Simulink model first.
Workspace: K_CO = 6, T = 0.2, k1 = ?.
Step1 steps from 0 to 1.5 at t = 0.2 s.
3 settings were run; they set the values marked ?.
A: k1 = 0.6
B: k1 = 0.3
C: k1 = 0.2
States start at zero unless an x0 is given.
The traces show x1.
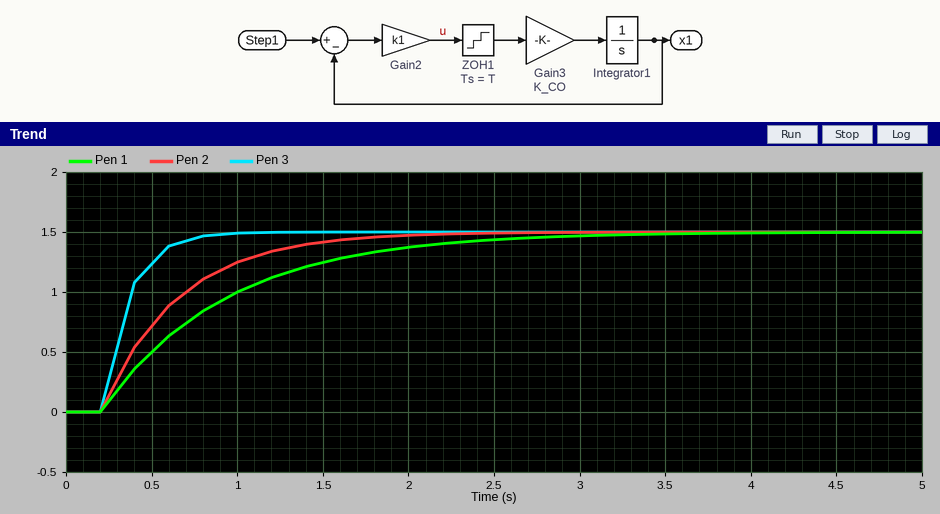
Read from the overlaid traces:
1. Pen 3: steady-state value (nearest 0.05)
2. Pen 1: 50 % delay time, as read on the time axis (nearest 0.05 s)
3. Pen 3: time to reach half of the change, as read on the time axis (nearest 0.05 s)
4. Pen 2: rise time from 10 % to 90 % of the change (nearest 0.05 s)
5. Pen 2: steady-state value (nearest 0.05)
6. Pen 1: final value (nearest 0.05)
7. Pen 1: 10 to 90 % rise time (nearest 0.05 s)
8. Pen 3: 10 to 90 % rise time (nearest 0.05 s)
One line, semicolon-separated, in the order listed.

1.50; 0.70 s; 0.35 s; 1.00 s; 1.50; 1.50; 1.60 s; 0.35 s
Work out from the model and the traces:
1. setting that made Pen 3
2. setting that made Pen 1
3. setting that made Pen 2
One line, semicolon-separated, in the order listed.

A; C; B
